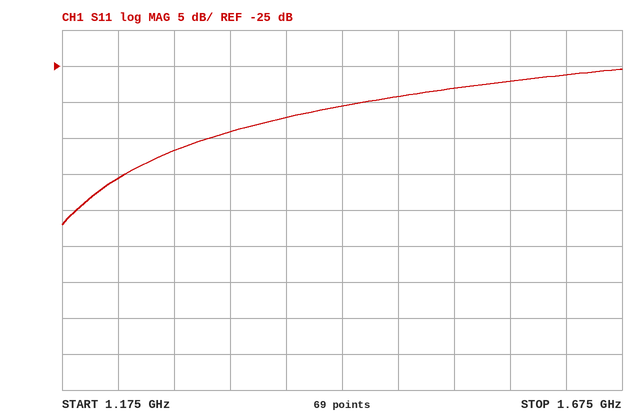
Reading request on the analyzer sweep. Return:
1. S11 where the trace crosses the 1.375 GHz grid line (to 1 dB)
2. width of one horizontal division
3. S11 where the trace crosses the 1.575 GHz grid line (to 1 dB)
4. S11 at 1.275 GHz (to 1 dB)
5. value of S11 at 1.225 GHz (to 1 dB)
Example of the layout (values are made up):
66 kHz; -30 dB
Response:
-32 dB; 50 MHz; -27 dB; -37 dB; -41 dB
